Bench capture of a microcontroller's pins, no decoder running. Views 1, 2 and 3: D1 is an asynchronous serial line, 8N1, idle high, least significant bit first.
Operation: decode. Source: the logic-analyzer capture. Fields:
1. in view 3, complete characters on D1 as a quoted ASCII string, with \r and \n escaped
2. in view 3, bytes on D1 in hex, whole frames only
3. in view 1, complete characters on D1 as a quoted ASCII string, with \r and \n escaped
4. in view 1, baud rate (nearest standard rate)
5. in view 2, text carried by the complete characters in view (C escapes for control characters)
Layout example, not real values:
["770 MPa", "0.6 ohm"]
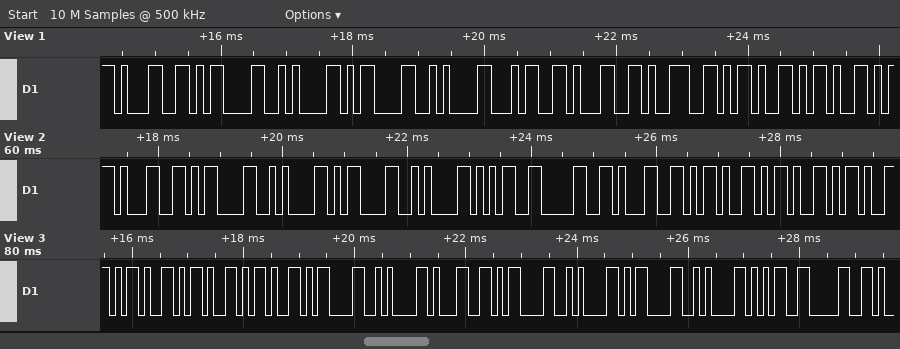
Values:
["\"---\\r\\n1\\r\\n\\r\\n50\"", "0x2D 0x2D 0x2D 0x0D 0x0A 0x31 0x0D 0x0A 0x0D 0x0A 0x35 0x30", "\"1\\r\\n\\r\\n419--\"", "9600 baud", "\"1\\r\\n\\r\\n501---\""]
